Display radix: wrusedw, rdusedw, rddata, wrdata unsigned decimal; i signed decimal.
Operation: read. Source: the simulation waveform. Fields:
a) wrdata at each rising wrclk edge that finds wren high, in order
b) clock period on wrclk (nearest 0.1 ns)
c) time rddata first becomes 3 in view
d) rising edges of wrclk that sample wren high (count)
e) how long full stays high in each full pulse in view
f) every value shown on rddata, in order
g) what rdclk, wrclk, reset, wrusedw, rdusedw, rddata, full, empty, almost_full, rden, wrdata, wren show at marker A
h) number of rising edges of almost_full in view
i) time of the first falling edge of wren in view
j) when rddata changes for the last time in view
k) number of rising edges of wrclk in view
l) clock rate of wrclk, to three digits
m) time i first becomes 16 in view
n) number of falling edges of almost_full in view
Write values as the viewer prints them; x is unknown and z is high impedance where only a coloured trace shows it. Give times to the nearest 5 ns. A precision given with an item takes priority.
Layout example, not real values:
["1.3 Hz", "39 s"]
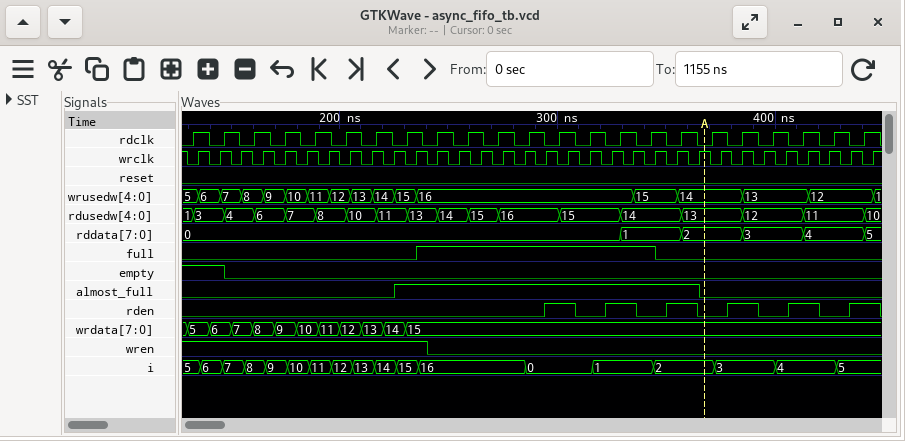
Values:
["5, 6, 7, 8, 9, 10, 11, 12, 13, 14, 15", "10 ns", "385 ns", "11", "110 ns", "0, 1, 2, 3, 4, 5", "rdclk=0, wrclk=1, reset=0, wrusedw=14, rdusedw=13, rddata=2, full=0, empty=0, almost_full=0, rden=0, wrdata=15, wren=0", "1", "240 ns", "440 ns", "32", "100 MHz", "235 ns", "1"]
